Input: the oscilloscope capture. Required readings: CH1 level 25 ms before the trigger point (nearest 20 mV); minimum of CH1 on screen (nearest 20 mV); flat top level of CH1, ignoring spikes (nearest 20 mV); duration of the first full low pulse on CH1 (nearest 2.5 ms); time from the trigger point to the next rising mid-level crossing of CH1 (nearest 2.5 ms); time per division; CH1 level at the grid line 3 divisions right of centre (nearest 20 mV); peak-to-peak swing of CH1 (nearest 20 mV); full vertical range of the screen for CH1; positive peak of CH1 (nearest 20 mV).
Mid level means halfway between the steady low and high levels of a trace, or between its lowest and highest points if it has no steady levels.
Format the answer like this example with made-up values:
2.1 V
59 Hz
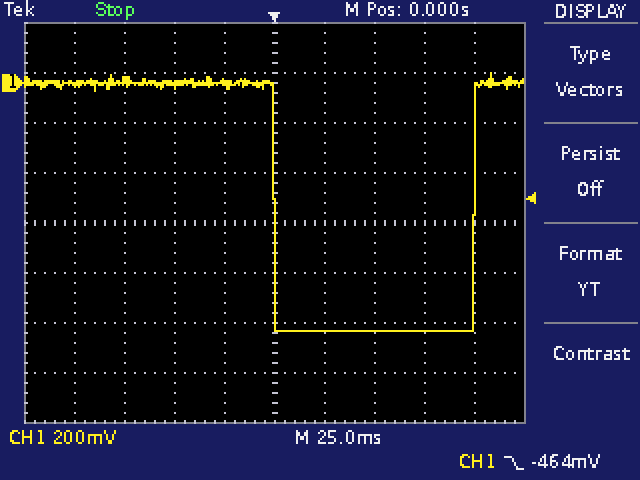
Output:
0 mV
-1.00 V
0 mV
100.0 ms
100.0 ms
25 ms
-1.00 V
1.04 V
1.6 V
40 mV
